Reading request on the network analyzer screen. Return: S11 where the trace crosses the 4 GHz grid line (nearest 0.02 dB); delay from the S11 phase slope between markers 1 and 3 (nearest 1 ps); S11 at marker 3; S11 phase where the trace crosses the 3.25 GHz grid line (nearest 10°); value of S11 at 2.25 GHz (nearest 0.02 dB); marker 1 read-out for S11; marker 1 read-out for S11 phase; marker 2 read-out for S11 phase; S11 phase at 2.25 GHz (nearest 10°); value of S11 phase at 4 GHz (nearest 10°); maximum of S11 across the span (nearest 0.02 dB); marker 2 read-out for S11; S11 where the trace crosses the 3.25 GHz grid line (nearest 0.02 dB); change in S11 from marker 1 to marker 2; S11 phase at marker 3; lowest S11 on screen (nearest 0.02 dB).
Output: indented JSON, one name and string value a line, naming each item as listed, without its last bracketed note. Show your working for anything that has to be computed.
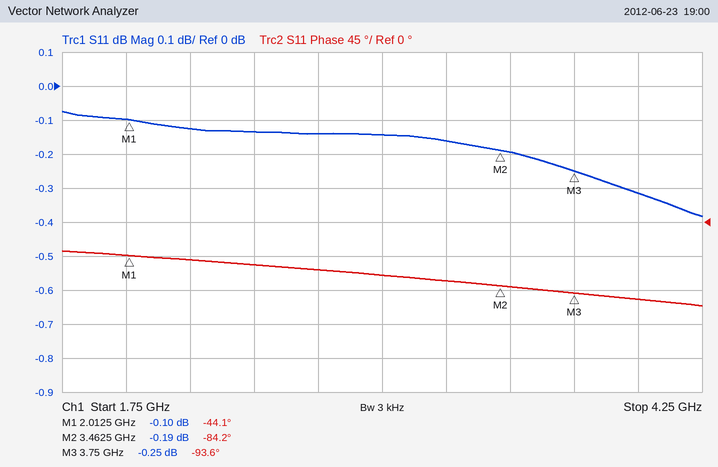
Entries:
{
  "S11 where the trace crosses the 4 GHz grid line": "-0.32 dB",
  "delay from the S11 phase slope between markers 1 and 3": "−(-93.6° − (-44.1°))/(360° × 1.7375 GHz) ≈ 79 ps",
  "S11 at marker 3": "-0.25 dB",
  "S11 phase where the trace crosses the 3.25 GHz grid line": "-80°",
  "value of S11 at 2.25 GHz": "-0.12 dB",
  "marker 1 read-out for S11": "-0.10 dB",
  "marker 1 read-out for S11 phase": "-44.1°",
  "marker 2 read-out for S11 phase": "-84.2°",
  "S11 phase at 2.25 GHz": "-50°",
  "value of S11 phase at 4 GHz": "-100°",
  "maximum of S11 across the span": "-0.08 dB",
  "marker 2 read-out for S11": "-0.19 dB",
  "S11 where the trace crosses the 3.25 GHz grid line": "-0.16 dB",
  "change in S11 from marker 1 to marker 2": "-0.19 − (-0.1) = -0.09 dB",
  "S11 phase at marker 3": "-93.6°",
  "lowest S11 on screen": "-0.38 dB"
}
